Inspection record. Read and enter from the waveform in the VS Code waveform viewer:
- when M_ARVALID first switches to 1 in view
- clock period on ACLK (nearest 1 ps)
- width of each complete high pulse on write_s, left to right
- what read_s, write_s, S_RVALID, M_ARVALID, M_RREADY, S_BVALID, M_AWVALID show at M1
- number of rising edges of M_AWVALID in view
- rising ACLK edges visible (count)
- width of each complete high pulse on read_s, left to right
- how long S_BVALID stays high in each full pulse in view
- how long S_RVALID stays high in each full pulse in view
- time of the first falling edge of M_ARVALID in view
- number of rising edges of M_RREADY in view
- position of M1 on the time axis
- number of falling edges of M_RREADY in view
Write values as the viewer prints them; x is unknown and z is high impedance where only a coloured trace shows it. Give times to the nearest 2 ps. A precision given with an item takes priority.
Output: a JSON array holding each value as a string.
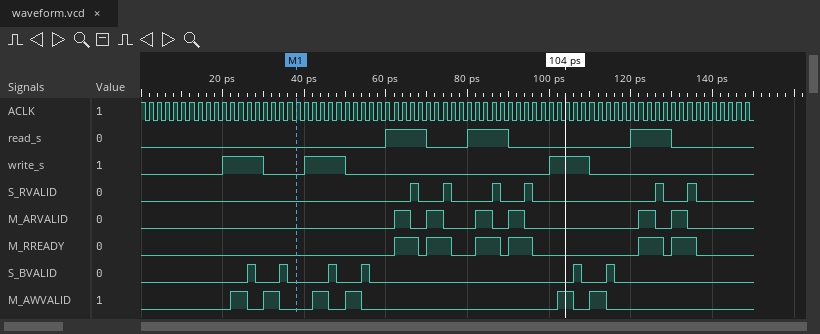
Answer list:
["62 ps", "2 ps", "10 ps, 10 ps, 10 ps", "read_s=0, write_s=0, S_RVALID=0, M_ARVALID=0, M_RREADY=0, S_BVALID=0, M_AWVALID=0", "6", "74", "10 ps, 10 ps, 10 ps", "2 ps, 2 ps, 2 ps, 2 ps, 2 ps, 2 ps", "2 ps, 2 ps, 2 ps, 2 ps, 2 ps, 2 ps", "66 ps", "6", "38 ps", "6"]
